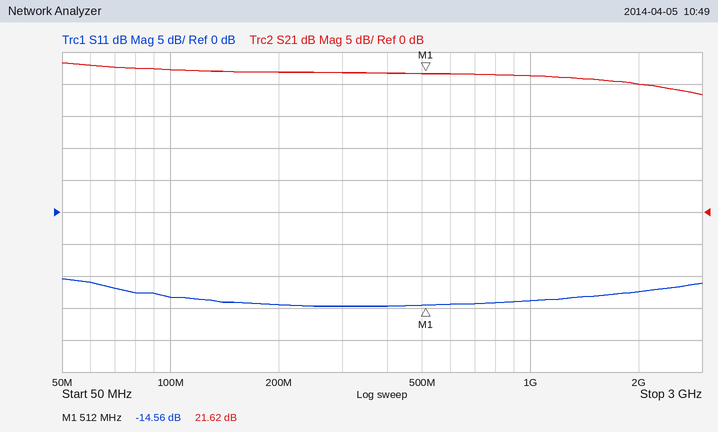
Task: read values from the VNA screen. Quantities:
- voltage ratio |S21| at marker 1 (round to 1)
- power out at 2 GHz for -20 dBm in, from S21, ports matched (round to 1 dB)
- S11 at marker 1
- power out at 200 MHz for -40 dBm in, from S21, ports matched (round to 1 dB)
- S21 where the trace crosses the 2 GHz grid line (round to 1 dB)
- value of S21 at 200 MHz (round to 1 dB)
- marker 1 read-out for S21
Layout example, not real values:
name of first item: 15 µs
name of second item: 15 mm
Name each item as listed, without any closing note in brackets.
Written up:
voltage ratio |S21| at marker 1: 12
power out at 2 GHz for -20 dBm in, from S21, ports matched: 0 dBm
S11 at marker 1: -14.56 dB
power out at 200 MHz for -40 dBm in, from S21, ports matched: -18 dBm
S21 where the trace crosses the 2 GHz grid line: 20 dB
value of S21 at 200 MHz: 22 dB
marker 1 read-out for S21: 21.62 dB
